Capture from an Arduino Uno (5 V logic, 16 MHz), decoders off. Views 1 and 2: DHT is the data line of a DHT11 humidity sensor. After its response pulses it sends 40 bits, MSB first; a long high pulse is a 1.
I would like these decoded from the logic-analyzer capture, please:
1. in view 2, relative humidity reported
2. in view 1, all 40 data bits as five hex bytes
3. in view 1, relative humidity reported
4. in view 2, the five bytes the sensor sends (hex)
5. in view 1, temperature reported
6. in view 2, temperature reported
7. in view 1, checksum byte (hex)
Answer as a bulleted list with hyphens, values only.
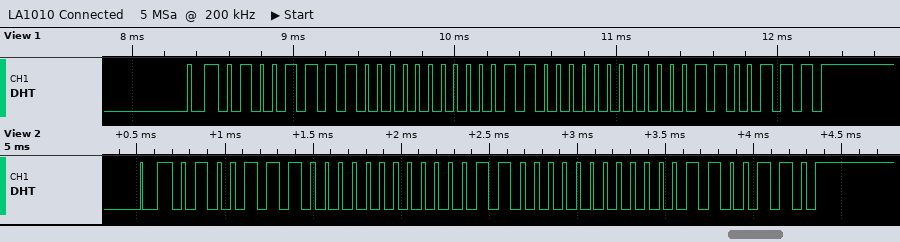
- 78 %
- 4F 00 18 00 67
- 79 %
- 4E 00 18 00 66
- 24.0 °C
- 24.0 °C
- 0x67
